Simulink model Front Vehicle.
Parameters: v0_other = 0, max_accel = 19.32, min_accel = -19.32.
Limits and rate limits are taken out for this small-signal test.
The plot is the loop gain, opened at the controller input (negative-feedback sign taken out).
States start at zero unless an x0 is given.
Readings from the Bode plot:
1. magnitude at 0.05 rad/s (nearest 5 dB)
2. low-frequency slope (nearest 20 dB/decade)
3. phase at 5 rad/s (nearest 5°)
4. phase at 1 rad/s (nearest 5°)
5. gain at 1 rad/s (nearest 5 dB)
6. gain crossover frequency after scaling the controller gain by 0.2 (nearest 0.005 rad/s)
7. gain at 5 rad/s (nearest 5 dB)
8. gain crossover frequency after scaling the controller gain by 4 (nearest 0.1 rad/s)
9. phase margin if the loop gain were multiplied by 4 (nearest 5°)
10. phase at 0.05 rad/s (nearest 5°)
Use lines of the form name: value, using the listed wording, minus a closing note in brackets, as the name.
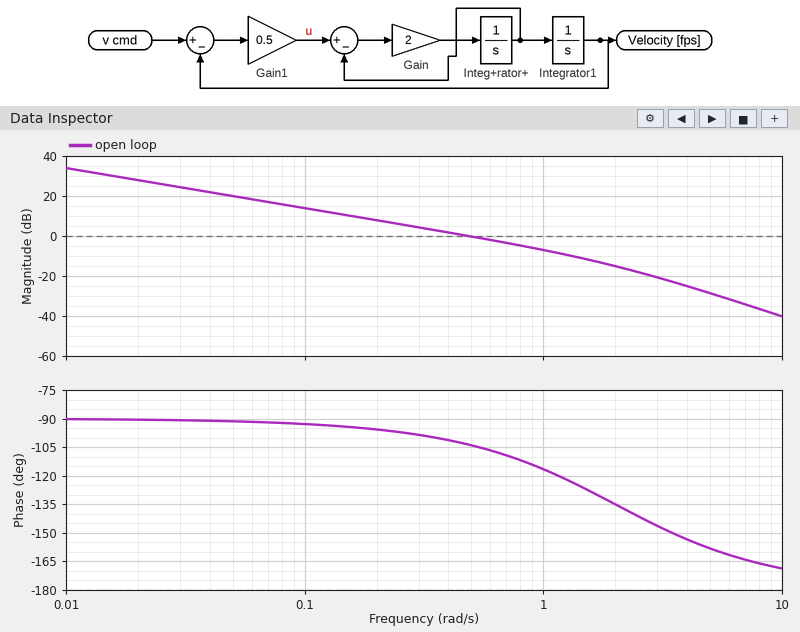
magnitude at 0.05 rad/s: 20 dB
low-frequency slope: -20 dB/decade
phase at 5 rad/s: -160°
phase at 1 rad/s: -115°
gain at 1 rad/s: -5 dB
gain crossover frequency after scaling the controller gain by 0.2: 0.100 rad/s
gain at 5 rad/s: -30 dB
gain crossover frequency after scaling the controller gain by 4: 1.6 rad/s
phase margin if the loop gain were multiplied by 4: 50°
phase at 0.05 rad/s: -90°
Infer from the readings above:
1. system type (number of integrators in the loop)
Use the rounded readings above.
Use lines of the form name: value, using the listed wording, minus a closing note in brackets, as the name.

system type: 1
